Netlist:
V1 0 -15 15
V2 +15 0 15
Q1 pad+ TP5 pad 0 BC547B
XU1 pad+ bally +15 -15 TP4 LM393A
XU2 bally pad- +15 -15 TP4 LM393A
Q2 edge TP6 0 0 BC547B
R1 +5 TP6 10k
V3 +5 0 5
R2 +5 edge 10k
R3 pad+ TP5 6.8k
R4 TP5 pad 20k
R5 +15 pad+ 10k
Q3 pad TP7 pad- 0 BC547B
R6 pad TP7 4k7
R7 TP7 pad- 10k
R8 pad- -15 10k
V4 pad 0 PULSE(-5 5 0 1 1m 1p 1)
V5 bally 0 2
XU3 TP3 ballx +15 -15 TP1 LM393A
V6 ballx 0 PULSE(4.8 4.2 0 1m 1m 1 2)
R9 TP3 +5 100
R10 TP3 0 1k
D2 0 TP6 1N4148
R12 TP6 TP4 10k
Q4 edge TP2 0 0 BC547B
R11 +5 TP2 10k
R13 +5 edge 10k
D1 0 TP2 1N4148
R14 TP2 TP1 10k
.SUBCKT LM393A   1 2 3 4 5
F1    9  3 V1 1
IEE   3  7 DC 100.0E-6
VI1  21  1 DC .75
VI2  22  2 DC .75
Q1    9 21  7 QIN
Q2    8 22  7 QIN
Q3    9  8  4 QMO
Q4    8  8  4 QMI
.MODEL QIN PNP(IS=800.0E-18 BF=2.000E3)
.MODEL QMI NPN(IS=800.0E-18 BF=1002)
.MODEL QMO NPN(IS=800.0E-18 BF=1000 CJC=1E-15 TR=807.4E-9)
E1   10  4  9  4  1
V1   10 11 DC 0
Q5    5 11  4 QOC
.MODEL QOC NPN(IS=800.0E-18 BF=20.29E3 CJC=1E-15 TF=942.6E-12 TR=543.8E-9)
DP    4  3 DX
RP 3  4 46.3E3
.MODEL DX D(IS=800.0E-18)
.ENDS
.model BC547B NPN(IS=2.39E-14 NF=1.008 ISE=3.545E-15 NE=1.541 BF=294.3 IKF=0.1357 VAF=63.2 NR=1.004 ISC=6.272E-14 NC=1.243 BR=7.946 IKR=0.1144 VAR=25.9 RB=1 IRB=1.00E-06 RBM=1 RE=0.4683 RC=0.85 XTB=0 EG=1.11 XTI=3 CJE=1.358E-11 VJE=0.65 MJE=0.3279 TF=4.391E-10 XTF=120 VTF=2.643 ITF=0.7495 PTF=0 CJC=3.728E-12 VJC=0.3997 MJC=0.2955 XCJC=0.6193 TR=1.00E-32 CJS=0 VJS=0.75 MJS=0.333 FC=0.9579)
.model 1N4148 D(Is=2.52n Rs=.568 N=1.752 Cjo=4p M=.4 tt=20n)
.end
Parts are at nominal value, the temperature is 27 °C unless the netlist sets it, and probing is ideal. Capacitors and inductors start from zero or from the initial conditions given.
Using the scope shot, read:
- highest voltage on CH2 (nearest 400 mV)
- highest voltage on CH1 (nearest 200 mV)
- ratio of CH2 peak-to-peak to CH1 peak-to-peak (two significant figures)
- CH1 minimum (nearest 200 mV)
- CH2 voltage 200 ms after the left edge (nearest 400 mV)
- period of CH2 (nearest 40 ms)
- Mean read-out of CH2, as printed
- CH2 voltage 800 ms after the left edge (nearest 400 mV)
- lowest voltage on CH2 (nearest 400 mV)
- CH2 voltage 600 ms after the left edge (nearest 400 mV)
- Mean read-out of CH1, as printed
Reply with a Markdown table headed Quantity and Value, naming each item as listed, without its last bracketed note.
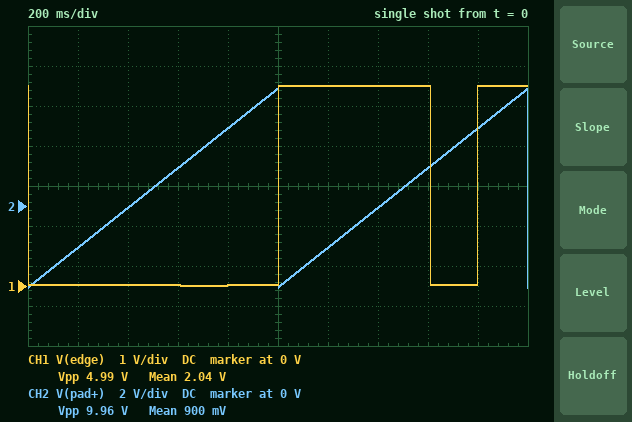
| Quantity | Value |
|---|---|
| highest voltage on CH2 | 6.0 V |
| highest voltage on CH1 | 5.0 V |
| ratio of CH2 peak-to-peak to CH1 peak-to-peak | 2.0 |
| CH1 minimum | 0 V |
| CH2 voltage 200 ms after the left edge | -2.0 V |
| period of CH2 | 1.00 s |
| Mean read-out of CH2, as printed | 900 mV |
| CH2 voltage 800 ms after the left edge | 4.0 V |
| lowest voltage on CH2 | -4.0 V |
| CH2 voltage 600 ms after the left edge | 2.0 V |
| Mean read-out of CH1, as printed | 2.04 V |
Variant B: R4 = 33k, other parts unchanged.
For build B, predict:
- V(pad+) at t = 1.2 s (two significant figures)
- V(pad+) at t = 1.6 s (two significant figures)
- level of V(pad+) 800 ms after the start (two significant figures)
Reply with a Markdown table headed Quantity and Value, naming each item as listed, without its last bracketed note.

| Quantity | Value |
|---|---|
| V(pad+) at t = 1.2 s | -2.2 V |
| V(pad+) at t = 1.6 s | 1.8 V |
| level of V(pad+) 800 ms after the start | 3.8 V |
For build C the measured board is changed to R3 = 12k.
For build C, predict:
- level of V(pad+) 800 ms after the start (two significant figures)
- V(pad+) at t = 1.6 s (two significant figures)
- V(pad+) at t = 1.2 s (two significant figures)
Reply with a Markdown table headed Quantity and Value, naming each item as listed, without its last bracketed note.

| Quantity | Value |
|---|---|
| level of V(pad+) 800 ms after the start | 4.1 V |
| V(pad+) at t = 1.6 s | 2.1 V |
| V(pad+) at t = 1.2 s | -1.9 V |
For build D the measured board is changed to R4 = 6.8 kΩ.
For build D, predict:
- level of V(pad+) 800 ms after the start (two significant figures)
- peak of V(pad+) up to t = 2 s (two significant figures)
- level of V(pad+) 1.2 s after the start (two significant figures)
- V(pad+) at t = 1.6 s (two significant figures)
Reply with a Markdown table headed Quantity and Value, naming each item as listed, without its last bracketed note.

| Quantity | Value |
|---|---|
| level of V(pad+) 800 ms after the start | 4.3 V |
| peak of V(pad+) up to t = 2 s | 6.3 V |
| level of V(pad+) 1.2 s after the start | -1.7 V |
| V(pad+) at t = 1.6 s | 2.3 V |
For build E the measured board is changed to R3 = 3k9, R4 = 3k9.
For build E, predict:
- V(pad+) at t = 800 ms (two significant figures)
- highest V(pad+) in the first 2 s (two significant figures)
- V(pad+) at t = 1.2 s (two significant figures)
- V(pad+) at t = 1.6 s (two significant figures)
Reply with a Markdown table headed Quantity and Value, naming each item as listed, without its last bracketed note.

| Quantity | Value |
|---|---|
| V(pad+) at t = 800 ms | 4.3 V |
| highest V(pad+) in the first 2 s | 6.3 V |
| V(pad+) at t = 1.2 s | -1.7 V |
| V(pad+) at t = 1.6 s | 2.3 V |
